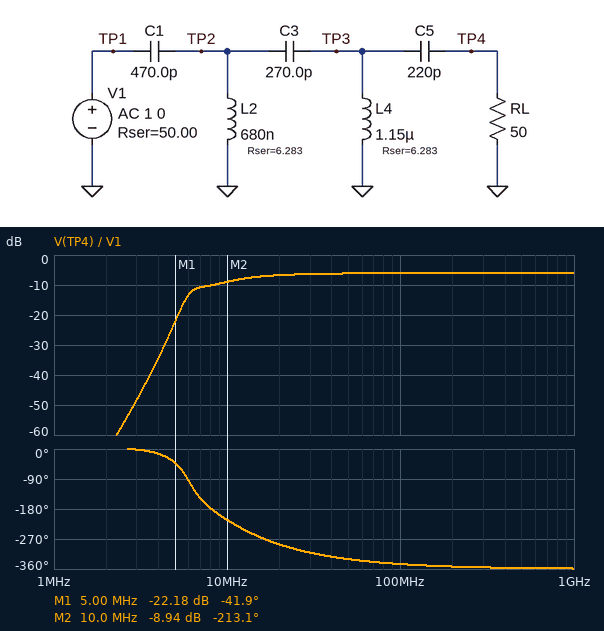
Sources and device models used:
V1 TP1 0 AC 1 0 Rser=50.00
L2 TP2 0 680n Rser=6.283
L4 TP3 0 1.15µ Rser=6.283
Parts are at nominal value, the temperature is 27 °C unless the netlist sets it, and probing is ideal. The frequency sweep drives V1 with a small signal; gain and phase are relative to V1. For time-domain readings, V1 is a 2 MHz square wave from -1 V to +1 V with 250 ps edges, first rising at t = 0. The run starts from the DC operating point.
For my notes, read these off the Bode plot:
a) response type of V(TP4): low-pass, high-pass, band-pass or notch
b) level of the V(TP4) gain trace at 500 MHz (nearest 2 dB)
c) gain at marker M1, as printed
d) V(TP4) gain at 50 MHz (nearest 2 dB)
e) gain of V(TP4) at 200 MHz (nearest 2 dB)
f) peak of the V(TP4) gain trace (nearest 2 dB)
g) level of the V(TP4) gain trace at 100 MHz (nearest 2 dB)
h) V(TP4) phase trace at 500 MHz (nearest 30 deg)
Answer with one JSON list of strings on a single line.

["high-pass", "-6 dB", "-22.18 dB", "-6 dB", "-6 dB", "-6 dB", "-6 dB", "-360 deg"]
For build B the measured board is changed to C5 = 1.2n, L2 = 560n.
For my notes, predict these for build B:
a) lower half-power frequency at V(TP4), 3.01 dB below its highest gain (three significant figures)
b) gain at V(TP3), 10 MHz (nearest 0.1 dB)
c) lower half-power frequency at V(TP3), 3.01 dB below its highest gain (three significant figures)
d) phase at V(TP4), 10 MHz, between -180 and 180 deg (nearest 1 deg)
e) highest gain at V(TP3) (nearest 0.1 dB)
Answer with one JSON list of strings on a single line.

["8.66 MHz", "-7.7 dB", "8.30 MHz", "128 deg", "-6.0 dB"]
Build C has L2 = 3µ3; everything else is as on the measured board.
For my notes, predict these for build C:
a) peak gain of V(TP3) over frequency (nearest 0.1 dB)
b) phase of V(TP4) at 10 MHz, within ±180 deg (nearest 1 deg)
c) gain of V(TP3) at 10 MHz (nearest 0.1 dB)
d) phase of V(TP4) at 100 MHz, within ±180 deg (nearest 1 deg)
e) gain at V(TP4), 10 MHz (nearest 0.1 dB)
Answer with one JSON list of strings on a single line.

["-1.5 dB", "110 deg", "-2.2 dB", "12 deg", "-7.1 dB"]
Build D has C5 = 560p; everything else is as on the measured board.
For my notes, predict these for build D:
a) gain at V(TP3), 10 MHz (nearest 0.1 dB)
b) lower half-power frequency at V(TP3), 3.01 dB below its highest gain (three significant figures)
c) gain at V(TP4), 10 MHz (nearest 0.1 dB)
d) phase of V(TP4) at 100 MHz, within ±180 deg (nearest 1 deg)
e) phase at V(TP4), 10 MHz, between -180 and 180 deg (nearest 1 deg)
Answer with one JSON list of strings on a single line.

["-6.4 dB", "6.29 MHz", "-7.6 dB", "12 deg", "128 deg"]
